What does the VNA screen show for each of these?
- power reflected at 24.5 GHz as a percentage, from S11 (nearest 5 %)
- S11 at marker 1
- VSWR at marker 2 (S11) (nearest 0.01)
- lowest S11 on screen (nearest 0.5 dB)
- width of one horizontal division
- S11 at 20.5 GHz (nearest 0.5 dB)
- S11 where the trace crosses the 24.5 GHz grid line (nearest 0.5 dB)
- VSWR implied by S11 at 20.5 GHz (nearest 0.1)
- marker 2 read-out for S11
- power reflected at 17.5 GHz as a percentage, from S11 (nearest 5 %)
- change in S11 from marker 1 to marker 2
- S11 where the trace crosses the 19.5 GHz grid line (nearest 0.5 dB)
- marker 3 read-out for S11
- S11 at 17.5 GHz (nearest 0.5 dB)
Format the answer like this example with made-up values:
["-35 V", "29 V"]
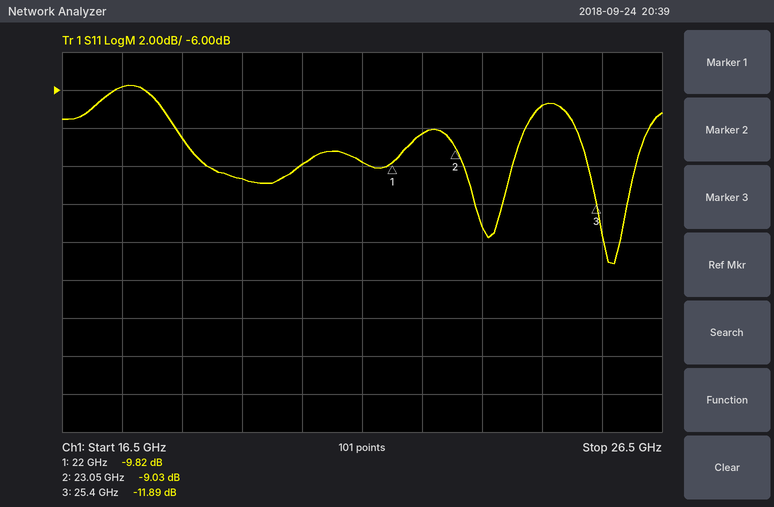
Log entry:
["20 %", "-9.82 dB", "2.09", "-15.0 dB", "1 GHz", "-10.0 dB", "-7.0 dB", "1.9", "-9.03 dB", "25 %", "0.79 dB", "-10.5 dB", "-11.89 dB", "-6.0 dB"]
